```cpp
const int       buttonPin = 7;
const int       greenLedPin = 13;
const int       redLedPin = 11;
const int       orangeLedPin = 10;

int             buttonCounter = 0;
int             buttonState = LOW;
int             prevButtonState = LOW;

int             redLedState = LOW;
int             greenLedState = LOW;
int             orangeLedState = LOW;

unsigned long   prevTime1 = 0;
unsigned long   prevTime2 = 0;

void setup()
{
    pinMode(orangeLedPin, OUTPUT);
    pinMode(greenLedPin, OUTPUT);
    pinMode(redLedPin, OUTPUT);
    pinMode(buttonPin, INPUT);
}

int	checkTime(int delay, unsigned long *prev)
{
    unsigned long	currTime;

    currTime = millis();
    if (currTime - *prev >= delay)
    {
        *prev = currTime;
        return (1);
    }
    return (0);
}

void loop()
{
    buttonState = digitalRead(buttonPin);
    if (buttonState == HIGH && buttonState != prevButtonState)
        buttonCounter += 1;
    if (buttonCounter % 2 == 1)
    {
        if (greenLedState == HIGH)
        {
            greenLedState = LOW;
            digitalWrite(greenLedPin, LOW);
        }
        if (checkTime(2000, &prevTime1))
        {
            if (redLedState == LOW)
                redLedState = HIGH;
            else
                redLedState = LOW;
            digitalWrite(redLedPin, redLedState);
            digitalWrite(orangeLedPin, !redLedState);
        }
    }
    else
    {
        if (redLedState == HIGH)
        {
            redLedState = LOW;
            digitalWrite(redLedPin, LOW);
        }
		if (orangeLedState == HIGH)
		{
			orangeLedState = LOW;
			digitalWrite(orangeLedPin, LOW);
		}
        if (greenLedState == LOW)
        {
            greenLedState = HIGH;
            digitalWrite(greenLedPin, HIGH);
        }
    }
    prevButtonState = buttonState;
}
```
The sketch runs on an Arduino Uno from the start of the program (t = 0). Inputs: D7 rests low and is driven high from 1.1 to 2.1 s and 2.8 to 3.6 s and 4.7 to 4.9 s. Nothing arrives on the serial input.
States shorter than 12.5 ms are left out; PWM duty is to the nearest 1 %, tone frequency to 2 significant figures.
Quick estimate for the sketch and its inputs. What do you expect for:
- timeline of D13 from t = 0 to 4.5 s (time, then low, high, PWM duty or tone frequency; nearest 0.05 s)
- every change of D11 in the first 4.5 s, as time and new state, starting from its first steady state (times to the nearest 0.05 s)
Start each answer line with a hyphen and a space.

- 0 s high; 1.1 s low; 2.8 s high
- 0 s low; 2 s high; 2.8 s low
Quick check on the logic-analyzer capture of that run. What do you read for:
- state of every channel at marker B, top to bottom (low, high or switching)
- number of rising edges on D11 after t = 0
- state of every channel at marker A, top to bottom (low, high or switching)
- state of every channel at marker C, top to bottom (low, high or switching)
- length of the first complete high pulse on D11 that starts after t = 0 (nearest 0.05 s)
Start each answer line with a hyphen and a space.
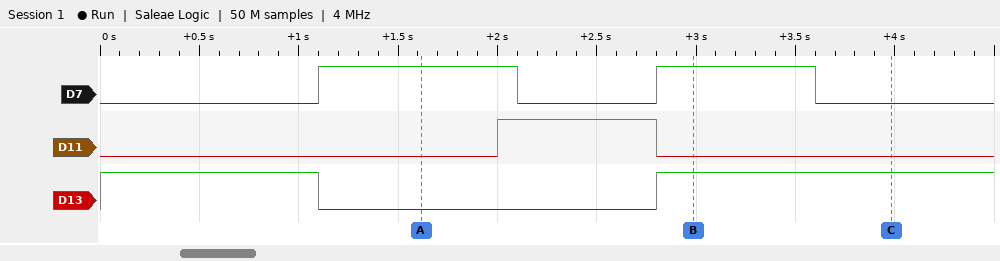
- D7 high, D11 low, D13 high
- 1
- D7 high, D11 low, D13 low
- D7 low, D11 low, D13 high
- 0.80 s
